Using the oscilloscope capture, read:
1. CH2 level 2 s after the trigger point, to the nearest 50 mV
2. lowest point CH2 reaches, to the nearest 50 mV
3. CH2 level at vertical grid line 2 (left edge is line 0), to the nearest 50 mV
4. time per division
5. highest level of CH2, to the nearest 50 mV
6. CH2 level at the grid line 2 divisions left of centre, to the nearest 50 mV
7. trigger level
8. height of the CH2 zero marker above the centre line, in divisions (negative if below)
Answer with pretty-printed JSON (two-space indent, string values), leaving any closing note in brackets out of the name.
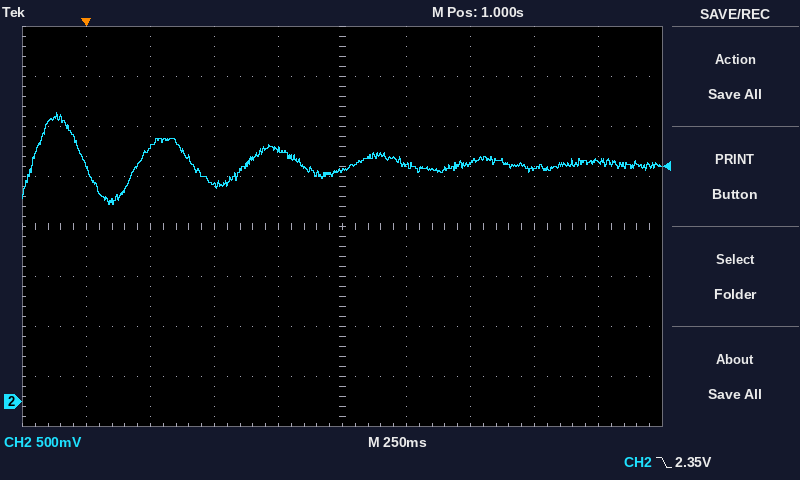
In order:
{
  "CH2 level 2 s after the trigger point, to the nearest 50 mV": "2.40 V",
  "lowest point CH2 reaches, to the nearest 50 mV": "1.95 V",
  "CH2 level at vertical grid line 2 (left edge is line 0), to the nearest 50 mV": "2.55 V",
  "time per division": "250 ms",
  "highest level of CH2, to the nearest 50 mV": "2.90 V",
  "CH2 level at the grid line 2 divisions left of centre, to the nearest 50 mV": "2.15 V",
  "trigger level": "2.35 V",
  "height of the CH2 zero marker above the centre line, in divisions": "-3.5 div"
}
